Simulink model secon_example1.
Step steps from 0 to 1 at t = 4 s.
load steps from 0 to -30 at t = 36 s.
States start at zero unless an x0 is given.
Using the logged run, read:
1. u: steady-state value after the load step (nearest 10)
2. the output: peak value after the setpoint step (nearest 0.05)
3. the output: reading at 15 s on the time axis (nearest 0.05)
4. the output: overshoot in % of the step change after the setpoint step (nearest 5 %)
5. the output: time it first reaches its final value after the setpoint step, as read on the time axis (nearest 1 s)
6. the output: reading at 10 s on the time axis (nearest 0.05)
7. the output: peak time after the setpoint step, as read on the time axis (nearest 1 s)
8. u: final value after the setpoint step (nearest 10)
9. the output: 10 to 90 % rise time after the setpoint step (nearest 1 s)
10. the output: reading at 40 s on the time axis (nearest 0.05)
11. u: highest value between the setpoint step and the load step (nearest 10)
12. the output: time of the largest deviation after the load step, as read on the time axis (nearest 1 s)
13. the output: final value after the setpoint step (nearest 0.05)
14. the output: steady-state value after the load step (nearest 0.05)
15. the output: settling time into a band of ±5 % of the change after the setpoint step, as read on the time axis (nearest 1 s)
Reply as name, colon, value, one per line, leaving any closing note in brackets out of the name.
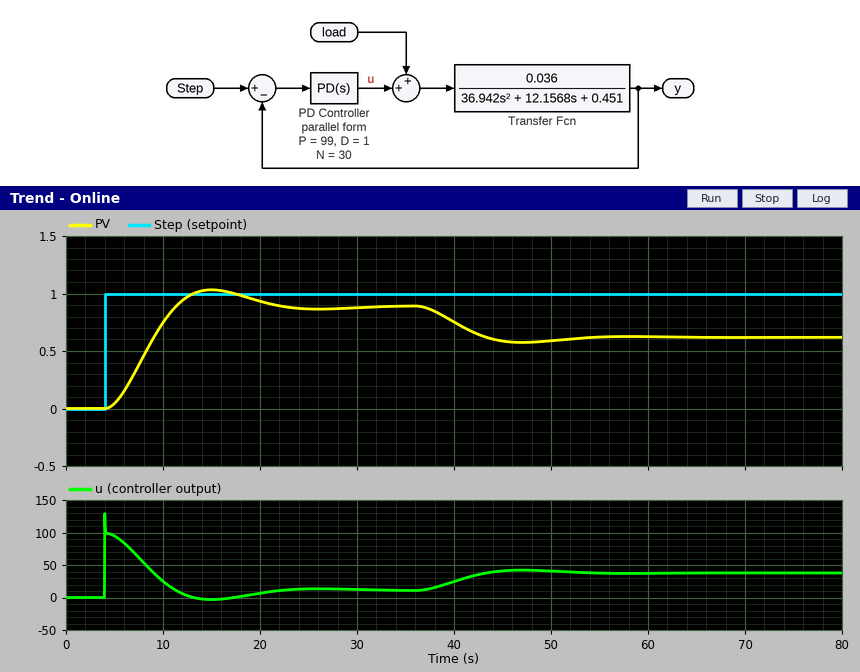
u: steady-state value after the load step: 40
the output: peak value after the setpoint step: 1.05
the output: reading at 15 s on the time axis: 1.05
the output: overshoot in % of the step change after the setpoint step: 15 %
the output: time it first reaches its final value after the setpoint step, as read on the time axis: 11 s
the output: reading at 10 s on the time axis: 0.75
the output: peak time after the setpoint step, as read on the time axis: 15 s
u: final value after the setpoint step: 10
the output: 10 to 90 % rise time after the setpoint step: 5 s
the output: reading at 40 s on the time axis: 0.75
u: highest value between the setpoint step and the load step: 130
the output: time of the largest deviation after the load step, as read on the time axis: 47 s
the output: final value after the setpoint step: 0.90
the output: steady-state value after the load step: 0.60
the output: settling time into a band of ±5 % of the change after the setpoint step, as read on the time axis: 20 s
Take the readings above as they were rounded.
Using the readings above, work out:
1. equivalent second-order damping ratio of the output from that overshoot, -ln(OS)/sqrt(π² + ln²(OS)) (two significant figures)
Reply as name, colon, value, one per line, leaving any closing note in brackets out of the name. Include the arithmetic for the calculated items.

equivalent second-order damping ratio of the output from that overshoot, -ln(OS)/sqrt(π² + ln²(OS)): ln(0.15) = -1.897; 1.897 / sqrt(9.870 + 3.599) = 0.52
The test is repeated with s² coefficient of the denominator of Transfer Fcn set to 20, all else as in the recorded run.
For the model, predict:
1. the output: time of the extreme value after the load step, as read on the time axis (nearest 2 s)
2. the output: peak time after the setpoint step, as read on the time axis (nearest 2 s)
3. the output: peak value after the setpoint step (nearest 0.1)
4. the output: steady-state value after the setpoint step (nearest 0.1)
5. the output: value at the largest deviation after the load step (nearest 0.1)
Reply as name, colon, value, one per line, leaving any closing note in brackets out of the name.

the output: time of the extreme value after the load step, as read on the time axis: 46 s
the output: peak time after the setpoint step, as read on the time axis: 14 s
the output: peak value after the setpoint step: 0.9
the output: steady-state value after the setpoint step: 0.9
the output: value at the largest deviation after the load step: 0.6
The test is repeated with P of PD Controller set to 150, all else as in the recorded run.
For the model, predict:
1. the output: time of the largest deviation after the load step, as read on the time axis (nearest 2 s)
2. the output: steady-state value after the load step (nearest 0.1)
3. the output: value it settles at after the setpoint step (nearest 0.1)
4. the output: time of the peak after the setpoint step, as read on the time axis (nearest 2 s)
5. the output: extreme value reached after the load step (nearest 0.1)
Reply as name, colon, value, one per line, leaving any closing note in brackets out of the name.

the output: time of the largest deviation after the load step, as read on the time axis: 44 s
the output: steady-state value after the load step: 0.7
the output: value it settles at after the setpoint step: 0.9
the output: time of the peak after the setpoint step, as read on the time axis: 12 s
the output: extreme value reached after the load step: 0.7
